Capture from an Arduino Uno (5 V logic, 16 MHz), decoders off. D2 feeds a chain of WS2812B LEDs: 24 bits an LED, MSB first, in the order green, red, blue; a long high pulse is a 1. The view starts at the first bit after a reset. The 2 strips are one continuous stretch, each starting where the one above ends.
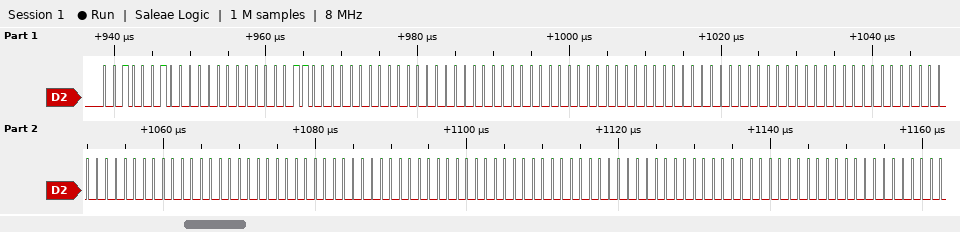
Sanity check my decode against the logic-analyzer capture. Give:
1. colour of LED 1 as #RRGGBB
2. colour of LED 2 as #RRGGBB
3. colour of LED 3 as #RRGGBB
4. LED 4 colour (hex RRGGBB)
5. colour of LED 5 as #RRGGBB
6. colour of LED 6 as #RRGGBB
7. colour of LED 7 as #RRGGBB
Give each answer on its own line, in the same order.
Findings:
#00220C
#000000
#000000
#000000
#000000
#000000
#000000
